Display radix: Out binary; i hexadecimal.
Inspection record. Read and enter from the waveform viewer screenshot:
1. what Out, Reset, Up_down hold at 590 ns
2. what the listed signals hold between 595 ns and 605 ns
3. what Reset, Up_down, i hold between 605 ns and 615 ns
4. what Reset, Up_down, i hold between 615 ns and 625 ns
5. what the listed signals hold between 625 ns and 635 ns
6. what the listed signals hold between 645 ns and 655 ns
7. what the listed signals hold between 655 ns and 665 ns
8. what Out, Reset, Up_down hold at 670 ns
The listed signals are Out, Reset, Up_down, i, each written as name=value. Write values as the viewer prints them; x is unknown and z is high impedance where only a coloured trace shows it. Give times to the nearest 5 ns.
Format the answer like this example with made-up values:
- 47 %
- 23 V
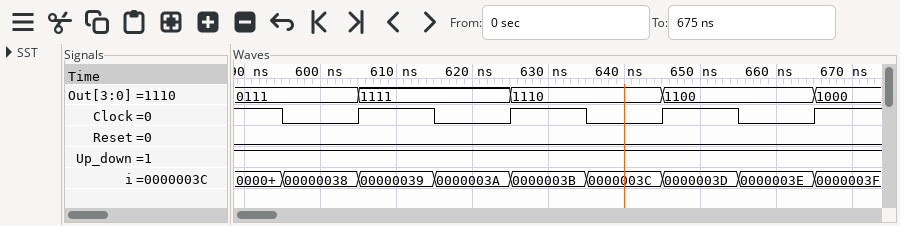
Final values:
- Out=0111, Reset=0, Up_down=1
- Out=0111, Reset=0, Up_down=1, i=00000038
- Reset=0, Up_down=1, i=00000039
- Reset=0, Up_down=1, i=0000003A
- Out=1110, Reset=0, Up_down=1, i=0000003B
- Out=1100, Reset=0, Up_down=1, i=0000003D
- Out=1100, Reset=0, Up_down=1, i=0000003E
- Out=1000, Reset=0, Up_down=1
